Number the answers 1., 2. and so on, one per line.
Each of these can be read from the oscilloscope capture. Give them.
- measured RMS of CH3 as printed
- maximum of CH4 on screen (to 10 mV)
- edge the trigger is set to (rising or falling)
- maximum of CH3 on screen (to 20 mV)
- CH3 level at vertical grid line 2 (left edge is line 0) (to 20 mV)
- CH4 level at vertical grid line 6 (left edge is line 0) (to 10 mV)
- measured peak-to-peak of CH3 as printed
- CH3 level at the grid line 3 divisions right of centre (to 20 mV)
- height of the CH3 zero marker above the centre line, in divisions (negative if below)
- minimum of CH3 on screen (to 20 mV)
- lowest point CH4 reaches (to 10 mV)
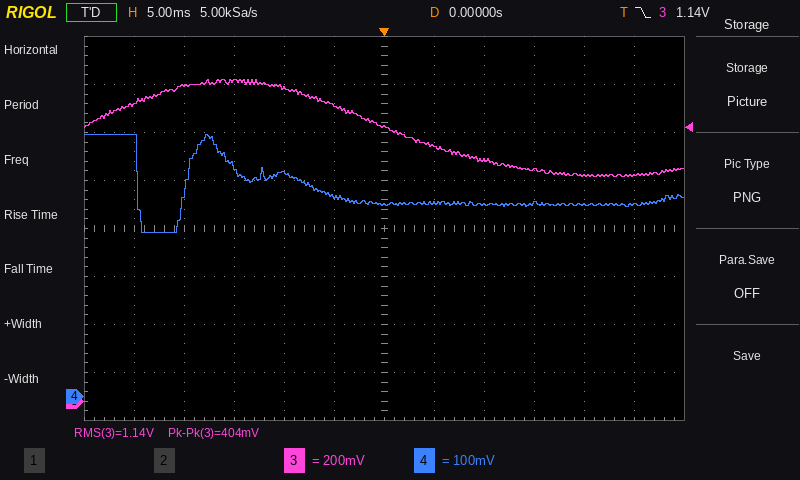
1. 1.14 V
2. 550 mV
3. falling
4. 1.34 V
5. 1.32 V
6. 400 mV
7. 404 mV
8. 960 mV
9. -3.6 div
10. 940 mV
11. 340 mV
